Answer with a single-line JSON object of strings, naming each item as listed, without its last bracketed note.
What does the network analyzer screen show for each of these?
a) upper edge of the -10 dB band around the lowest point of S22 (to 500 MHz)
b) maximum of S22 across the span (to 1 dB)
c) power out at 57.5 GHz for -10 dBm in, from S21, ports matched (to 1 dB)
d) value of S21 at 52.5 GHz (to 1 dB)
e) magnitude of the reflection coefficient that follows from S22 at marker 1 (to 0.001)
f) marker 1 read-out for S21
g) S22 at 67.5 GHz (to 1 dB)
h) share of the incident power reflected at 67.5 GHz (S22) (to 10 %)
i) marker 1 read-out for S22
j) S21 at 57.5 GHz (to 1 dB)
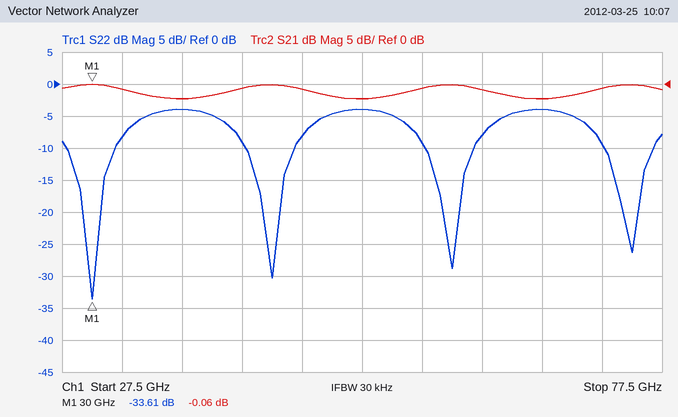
{"upper edge of the -10 dB band around the lowest point of S22": "32.0 GHz", "maximum of S22 across the span": "-4 dB", "power out at 57.5 GHz for -10 dBm in, from S21, ports matched": "-11 dBm", "value of S21 at 52.5 GHz": "-2 dB", "magnitude of the reflection coefficient that follows from S22 at marker 1": "0.021", "marker 1 read-out for S21": "-0.06 dB", "S22 at 67.5 GHz": "-4 dB", "share of the incident power reflected at 67.5 GHz (S22)": "40 %", "marker 1 read-out for S22": "-33.61 dB", "S21 at 57.5 GHz": "-1 dB"}
